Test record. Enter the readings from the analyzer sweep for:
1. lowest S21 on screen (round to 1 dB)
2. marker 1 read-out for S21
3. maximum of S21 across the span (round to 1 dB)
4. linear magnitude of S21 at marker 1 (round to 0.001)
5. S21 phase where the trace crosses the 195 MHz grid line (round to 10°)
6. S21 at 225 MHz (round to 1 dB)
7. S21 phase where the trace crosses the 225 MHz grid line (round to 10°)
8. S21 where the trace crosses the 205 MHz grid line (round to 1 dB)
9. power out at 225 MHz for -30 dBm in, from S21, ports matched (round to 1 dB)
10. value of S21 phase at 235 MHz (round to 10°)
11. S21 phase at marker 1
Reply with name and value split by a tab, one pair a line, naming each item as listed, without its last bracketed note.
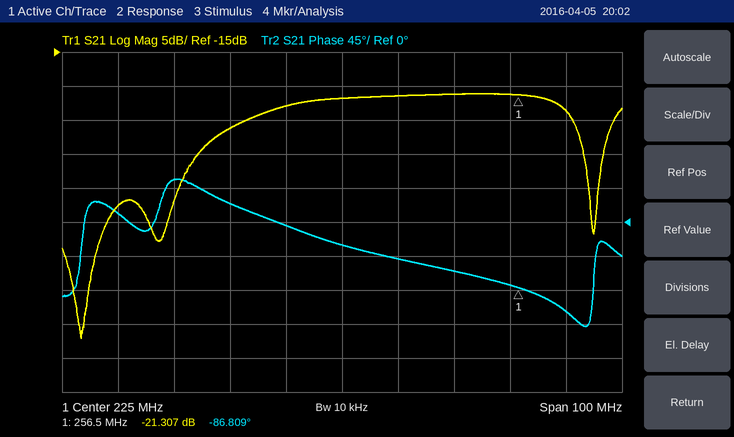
lowest S21 on screen	-57 dB
marker 1 read-out for S21	-21.307 dB
maximum of S21 across the span	-21 dB
linear magnitude of S21 at marker 1	0.086
S21 phase where the trace crosses the 195 MHz grid line	60°
S21 at 225 MHz	-22 dB
S21 phase where the trace crosses the 225 MHz grid line	-30°
S21 where the trace crosses the 205 MHz grid line	-26 dB
power out at 225 MHz for -30 dBm in, from S21, ports matched	-52 dBm
value of S21 phase at 235 MHz	-50°
S21 phase at marker 1	-86.809°
